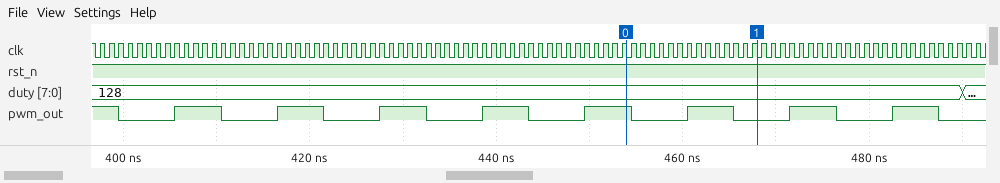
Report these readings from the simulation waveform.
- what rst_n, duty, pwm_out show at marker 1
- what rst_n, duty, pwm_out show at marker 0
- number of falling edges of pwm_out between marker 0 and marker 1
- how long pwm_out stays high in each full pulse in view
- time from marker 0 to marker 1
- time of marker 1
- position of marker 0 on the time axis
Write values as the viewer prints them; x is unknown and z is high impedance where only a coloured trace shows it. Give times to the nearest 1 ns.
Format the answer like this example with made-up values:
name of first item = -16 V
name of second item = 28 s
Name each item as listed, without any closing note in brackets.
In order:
what rst_n, duty, pwm_out show at marker 1 = rst_n=1, duty=128, pwm_out=0
what rst_n, duty, pwm_out show at marker 0 = rst_n=1, duty=128, pwm_out=1
number of falling edges of pwm_out between marker 0 and marker 1 = 2
how long pwm_out stays high in each full pulse in view = 5 ns, 5 ns, 5 ns, 5 ns, 5 ns, 5 ns, 5 ns, 5 ns
time from marker 0 to marker 1 = 14 ns
time of marker 1 = 468 ns
position of marker 0 on the time axis = 454 ns
